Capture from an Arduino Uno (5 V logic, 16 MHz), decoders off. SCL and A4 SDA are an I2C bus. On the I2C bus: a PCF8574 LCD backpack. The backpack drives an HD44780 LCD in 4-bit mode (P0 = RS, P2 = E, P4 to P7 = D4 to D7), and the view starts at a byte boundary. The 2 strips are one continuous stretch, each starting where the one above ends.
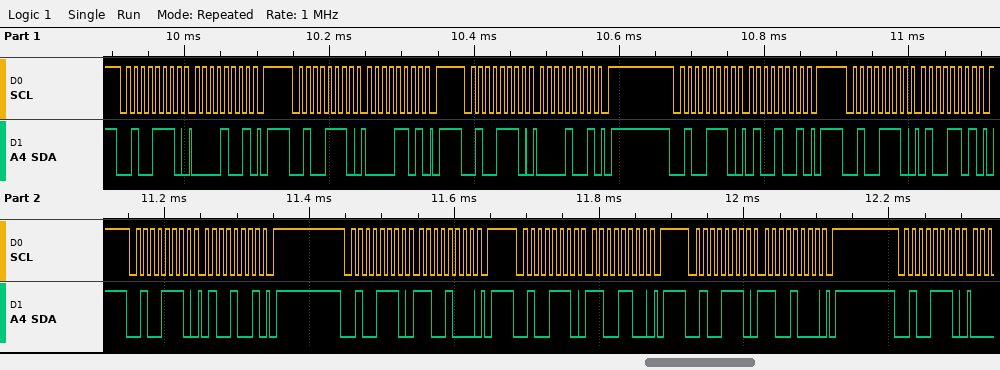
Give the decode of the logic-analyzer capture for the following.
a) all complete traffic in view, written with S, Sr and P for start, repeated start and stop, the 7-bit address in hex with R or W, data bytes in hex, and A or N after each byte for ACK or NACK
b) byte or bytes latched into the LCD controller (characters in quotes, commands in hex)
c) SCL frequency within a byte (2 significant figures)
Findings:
S 27W A 09 A P S 27W A 0D A P S 27W A 09 A P S 27W A 49 A P S 27W A 4D A P S 27W A 49 A P S 27W A C8 A P S 27W A CC A P S 27W A C8 A P S 27W A
data 0x04
100 kHz
